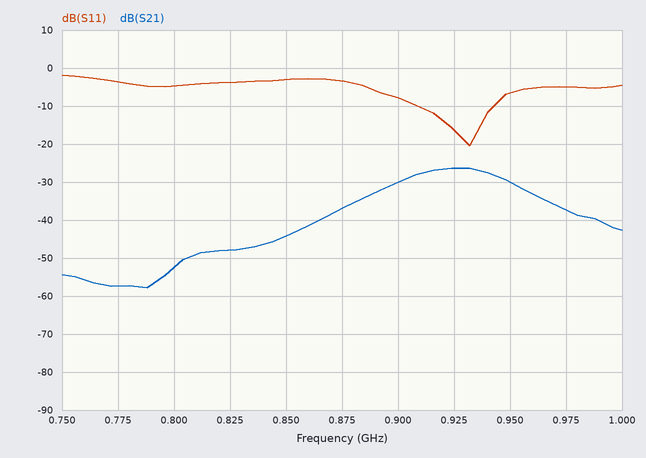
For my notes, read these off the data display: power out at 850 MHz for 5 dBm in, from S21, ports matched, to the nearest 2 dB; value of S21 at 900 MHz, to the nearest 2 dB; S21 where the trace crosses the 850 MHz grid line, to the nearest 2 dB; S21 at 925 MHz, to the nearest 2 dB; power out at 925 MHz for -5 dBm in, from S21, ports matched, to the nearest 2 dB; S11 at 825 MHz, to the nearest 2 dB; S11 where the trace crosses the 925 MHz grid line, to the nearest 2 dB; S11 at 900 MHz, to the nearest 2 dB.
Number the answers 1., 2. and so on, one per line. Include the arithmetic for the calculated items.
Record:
1. 5 dBm + (-44 dB) = -40 dBm
2. -30 dB
3. -44 dB
4. -26 dB
5. -5 dBm + (-26 dB) = -32 dBm
6. -4 dB
7. -16 dB
8. -8 dB
